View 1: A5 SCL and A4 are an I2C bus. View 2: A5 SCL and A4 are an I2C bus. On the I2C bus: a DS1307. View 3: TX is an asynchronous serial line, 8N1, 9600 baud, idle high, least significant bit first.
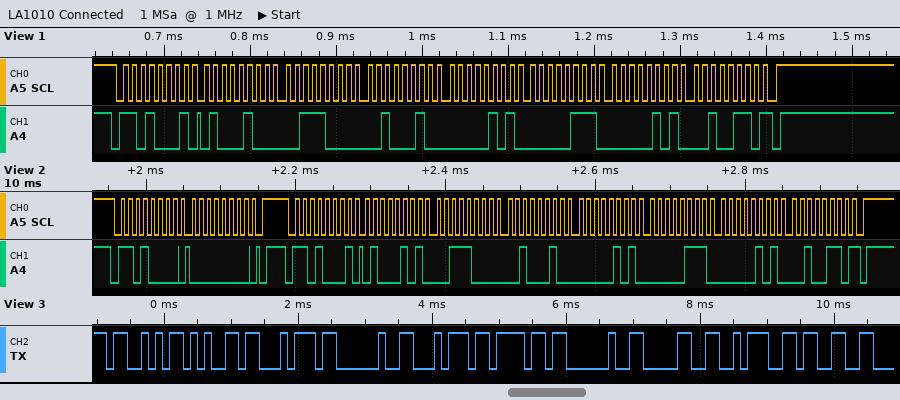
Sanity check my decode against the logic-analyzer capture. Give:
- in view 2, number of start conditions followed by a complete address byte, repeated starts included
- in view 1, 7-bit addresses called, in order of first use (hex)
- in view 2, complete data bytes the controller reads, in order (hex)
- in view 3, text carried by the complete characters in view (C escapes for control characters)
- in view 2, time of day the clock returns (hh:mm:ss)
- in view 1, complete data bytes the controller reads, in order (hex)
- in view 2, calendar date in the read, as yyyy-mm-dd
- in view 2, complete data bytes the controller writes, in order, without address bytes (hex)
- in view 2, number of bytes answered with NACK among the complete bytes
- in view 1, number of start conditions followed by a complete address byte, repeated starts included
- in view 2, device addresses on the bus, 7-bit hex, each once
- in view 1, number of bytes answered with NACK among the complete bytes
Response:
2
0x68
45 38 22 05 07 05 26
"Set to 0:3"
22:38:45
44 38 22 05 07 05 26
2026-05-07
00
1
1
0x68
1
